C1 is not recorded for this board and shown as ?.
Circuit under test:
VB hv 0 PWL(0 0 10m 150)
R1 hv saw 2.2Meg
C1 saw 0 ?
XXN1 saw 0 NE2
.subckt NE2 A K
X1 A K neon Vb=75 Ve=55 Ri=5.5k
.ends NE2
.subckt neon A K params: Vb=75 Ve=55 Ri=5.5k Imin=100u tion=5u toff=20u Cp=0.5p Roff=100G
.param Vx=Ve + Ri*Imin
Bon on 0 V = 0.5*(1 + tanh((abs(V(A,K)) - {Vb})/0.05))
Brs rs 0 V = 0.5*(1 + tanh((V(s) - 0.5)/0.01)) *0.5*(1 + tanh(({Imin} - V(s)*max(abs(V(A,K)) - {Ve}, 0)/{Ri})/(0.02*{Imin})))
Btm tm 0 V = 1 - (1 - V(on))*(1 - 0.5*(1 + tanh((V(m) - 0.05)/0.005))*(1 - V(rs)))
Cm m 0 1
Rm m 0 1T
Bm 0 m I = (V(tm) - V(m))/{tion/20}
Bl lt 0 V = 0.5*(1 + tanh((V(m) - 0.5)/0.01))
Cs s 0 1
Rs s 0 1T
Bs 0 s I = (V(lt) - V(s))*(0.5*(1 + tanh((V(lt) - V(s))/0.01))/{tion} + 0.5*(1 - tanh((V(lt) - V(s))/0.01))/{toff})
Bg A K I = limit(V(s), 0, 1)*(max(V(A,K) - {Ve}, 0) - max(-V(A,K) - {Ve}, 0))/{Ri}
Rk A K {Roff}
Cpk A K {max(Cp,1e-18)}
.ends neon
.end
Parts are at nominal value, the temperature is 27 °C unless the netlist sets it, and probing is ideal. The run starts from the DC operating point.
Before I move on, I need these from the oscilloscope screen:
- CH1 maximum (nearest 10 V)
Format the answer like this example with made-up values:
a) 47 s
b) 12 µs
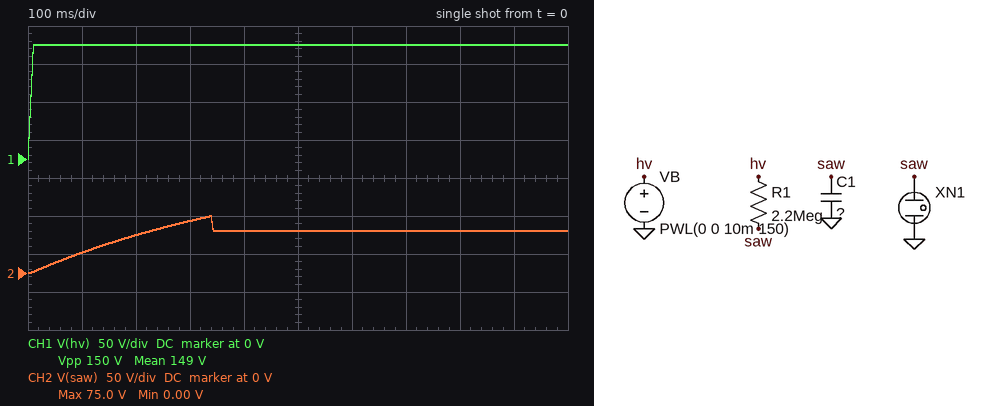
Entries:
a) 150 V
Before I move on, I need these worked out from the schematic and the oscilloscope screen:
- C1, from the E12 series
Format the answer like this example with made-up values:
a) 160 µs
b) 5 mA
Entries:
a) 220 nF
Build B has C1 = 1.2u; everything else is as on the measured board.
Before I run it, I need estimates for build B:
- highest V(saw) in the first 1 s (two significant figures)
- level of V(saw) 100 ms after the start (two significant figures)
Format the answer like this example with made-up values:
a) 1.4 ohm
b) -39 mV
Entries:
a) 47 V
b) 5.3 V
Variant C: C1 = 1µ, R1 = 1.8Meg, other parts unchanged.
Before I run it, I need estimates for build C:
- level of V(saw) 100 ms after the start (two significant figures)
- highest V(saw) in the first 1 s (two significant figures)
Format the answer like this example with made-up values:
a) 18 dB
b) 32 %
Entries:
a) 7.7 V
b) 64 V
